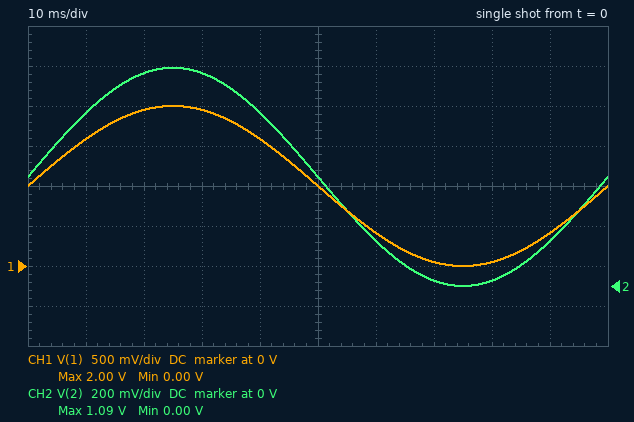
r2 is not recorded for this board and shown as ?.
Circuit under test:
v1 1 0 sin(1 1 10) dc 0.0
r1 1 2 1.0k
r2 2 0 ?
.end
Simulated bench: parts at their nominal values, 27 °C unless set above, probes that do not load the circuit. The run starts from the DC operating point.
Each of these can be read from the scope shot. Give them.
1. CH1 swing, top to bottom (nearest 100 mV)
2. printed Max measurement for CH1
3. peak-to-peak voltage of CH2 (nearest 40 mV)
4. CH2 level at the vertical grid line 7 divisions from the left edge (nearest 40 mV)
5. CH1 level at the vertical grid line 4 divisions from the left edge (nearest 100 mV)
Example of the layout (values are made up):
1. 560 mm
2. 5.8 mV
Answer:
1. 2.0 V
2. 2.00 V
3. 1.08 V
4. 40 mV
5. 1.6 V
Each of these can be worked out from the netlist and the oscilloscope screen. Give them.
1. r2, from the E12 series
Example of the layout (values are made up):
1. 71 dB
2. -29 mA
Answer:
1. 1.2 kΩ
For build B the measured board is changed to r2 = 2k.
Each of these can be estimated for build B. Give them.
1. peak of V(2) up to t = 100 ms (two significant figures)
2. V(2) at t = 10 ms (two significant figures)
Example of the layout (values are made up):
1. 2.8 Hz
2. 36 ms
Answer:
1. 1.3 V
2. 1.1 V
